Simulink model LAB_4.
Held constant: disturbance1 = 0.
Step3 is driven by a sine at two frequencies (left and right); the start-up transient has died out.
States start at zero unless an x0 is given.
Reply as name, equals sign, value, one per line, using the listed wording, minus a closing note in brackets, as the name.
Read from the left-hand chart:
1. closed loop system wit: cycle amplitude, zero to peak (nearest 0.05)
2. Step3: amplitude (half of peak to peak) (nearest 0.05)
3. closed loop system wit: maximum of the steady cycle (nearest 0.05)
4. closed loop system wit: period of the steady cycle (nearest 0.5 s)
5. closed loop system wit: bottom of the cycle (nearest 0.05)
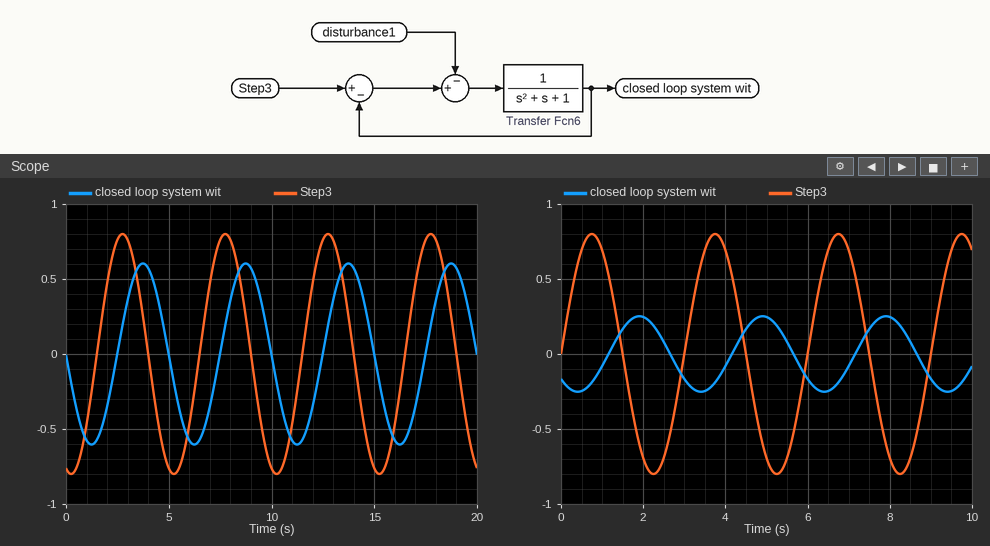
closed loop system wit: cycle amplitude, zero to peak = 0.60
Step3: amplitude (half of peak to peak) = 0.80
closed loop system wit: maximum of the steady cycle = 0.60
closed loop system wit: period of the steady cycle = 5.0 s
closed loop system wit: bottom of the cycle = -0.60
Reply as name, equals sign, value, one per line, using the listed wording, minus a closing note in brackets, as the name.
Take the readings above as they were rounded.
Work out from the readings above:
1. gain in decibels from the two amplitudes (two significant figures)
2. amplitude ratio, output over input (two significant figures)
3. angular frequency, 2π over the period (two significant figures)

gain in decibels from the two amplitudes = -2.5 dB
amplitude ratio, output over input = 0.75
angular frequency, 2π over the period = 1.3 rad/s
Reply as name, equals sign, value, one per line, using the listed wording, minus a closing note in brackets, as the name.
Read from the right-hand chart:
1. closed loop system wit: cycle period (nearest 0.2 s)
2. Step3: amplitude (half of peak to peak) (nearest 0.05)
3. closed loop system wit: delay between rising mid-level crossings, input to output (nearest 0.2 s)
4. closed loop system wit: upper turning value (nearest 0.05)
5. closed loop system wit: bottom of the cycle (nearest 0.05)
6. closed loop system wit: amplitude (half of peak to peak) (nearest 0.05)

closed loop system wit: cycle period = 3.0 s
Step3: amplitude (half of peak to peak) = 0.80
closed loop system wit: delay between rising mid-level crossings, input to output = 1.2 s
closed loop system wit: upper turning value = 0.25
closed loop system wit: bottom of the cycle = -0.25
closed loop system wit: amplitude (half of peak to peak) = 0.25
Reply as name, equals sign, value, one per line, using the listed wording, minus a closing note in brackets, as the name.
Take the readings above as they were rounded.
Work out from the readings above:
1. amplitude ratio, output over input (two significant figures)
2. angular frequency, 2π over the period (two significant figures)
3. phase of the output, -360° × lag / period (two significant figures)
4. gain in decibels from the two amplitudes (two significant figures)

amplitude ratio, output over input = 0.31
angular frequency, 2π over the period = 2.1 rad/s
phase of the output, -360° × lag / period = -140°
gain in decibels from the two amplitudes = -10 dB
